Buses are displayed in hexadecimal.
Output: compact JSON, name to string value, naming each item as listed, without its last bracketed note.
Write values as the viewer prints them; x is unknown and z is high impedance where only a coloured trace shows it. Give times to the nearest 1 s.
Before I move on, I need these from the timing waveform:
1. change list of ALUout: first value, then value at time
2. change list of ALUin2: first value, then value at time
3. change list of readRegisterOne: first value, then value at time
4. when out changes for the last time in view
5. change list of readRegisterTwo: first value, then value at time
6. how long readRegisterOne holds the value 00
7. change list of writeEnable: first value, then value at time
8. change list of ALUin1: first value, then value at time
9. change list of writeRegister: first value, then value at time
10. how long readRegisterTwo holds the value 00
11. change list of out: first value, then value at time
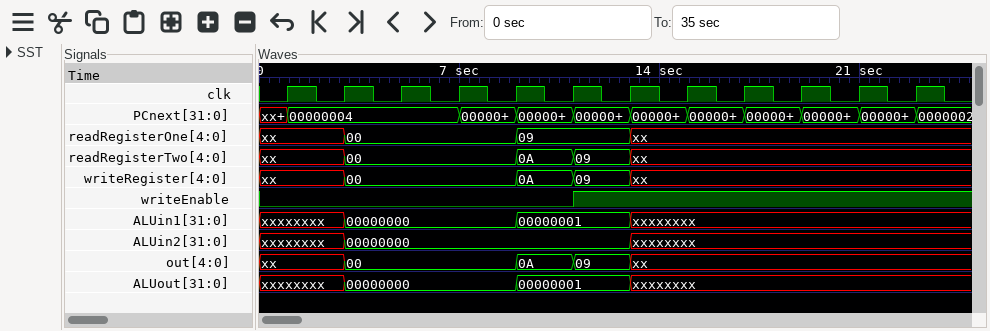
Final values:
{"change list of ALUout: first value, then value at time": "xxxxxxxx, 00000000 at 3 s, 00000001 at 9 s, xxxxxxxx at 13 s", "change list of ALUin2: first value, then value at time": "xxxxxxxx, 00000000 at 3 s, xxxxxxxx at 13 s", "change list of readRegisterOne: first value, then value at time": "xx, 00 at 3 s, 09 at 9 s, xx at 13 s", "when out changes for the last time in view": "13 s", "change list of readRegisterTwo: first value, then value at time": "xx, 00 at 3 s, 0A at 9 s, 09 at 11 s, xx at 13 s", "how long readRegisterOne holds the value 00": "6 s", "change list of writeEnable: first value, then value at time": "0, 1 at 11 s", "change list of ALUin1: first value, then value at time": "xxxxxxxx, 00000000 at 3 s, 00000001 at 9 s, xxxxxxxx at 13 s", "change list of writeRegister: first value, then value at time": "xx, 00 at 3 s, 0A at 9 s, 09 at 11 s, xx at 13 s", "how long readRegisterTwo holds the value 00": "6 s", "change list of out: first value, then value at time": "xx, 00 at 3 s, 0A at 9 s, 09 at 11 s, xx at 13 s"}
